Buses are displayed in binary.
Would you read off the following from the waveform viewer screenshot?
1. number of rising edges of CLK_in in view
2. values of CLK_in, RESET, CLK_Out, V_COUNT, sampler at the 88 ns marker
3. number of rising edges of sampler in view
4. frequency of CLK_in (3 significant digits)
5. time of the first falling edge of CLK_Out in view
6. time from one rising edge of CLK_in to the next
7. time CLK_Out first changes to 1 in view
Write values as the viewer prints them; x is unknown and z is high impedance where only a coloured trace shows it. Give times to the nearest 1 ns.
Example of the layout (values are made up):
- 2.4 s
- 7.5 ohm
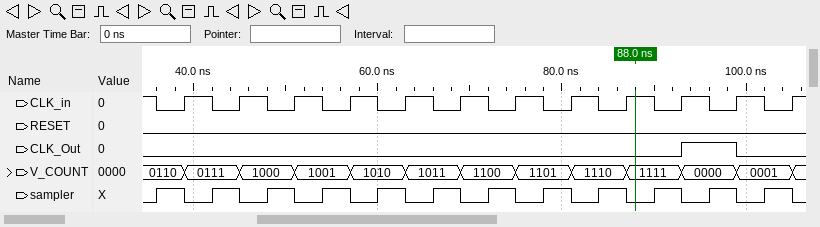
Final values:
- 12
- CLK_in=1, RESET=0, CLK_Out=0, V_COUNT=1111, sampler=0
- 12
- 167 MHz
- 99 ns
- 6 ns
- 93 ns
